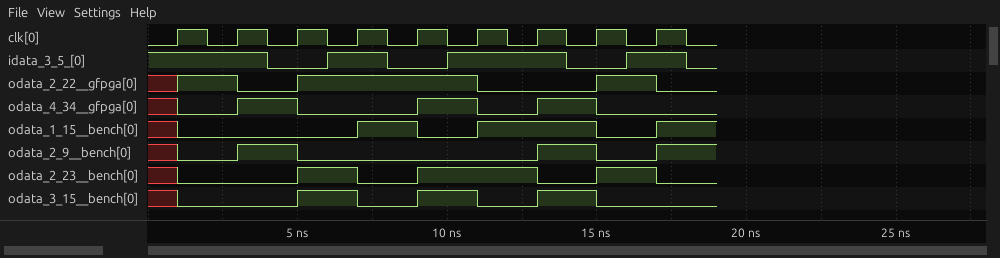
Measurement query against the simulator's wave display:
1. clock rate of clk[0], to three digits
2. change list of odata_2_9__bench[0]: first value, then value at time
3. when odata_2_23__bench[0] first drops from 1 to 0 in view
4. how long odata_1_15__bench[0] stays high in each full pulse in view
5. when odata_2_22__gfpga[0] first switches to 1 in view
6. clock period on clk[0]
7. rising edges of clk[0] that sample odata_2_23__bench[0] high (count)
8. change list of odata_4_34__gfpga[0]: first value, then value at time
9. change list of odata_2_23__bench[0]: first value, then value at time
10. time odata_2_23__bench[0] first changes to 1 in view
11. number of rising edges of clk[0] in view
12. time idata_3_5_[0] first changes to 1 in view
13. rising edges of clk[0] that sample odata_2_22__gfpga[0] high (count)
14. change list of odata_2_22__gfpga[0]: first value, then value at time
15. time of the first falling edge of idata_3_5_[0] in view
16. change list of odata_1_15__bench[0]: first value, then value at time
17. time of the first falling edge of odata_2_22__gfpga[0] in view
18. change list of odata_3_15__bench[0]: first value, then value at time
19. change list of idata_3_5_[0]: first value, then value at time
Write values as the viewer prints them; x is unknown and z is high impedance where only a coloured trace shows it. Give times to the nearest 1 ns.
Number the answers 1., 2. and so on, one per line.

1. 500 MHz
2. x, 0 at 1 ns, 1 at 3 ns, 0 at 5 ns, 1 at 13 ns, 0 at 15 ns, 1 at 17 ns
3. 7 ns
4. 2 ns, 4 ns
5. 1 ns
6. 2 ns
7. 4
8. x, 0 at 1 ns, 1 at 3 ns, 0 at 5 ns, 1 at 9 ns, 0 at 11 ns, 1 at 13 ns, 0 at 15 ns
9. x, 0 at 1 ns, 1 at 5 ns, 0 at 7 ns, 1 at 9 ns, 0 at 13 ns, 1 at 15 ns, 0 at 17 ns
10. 5 ns
11. 9
12. 6 ns
13. 5
14. x, 1 at 1 ns, 0 at 3 ns, 1 at 5 ns, 0 at 11 ns, 1 at 15 ns, 0 at 17 ns
15. 4 ns
16. x, 0 at 1 ns, 1 at 7 ns, 0 at 9 ns, 1 at 11 ns, 0 at 15 ns, 1 at 17 ns
17. 3 ns
18. x, 0 at 1 ns, 1 at 5 ns, 0 at 7 ns, 1 at 9 ns, 0 at 11 ns, 1 at 13 ns, 0 at 15 ns
19. 1, 0 at 4 ns, 1 at 6 ns, 0 at 8 ns, 1 at 10 ns, 0 at 14 ns, 1 at 16 ns, 0 at 18 ns
